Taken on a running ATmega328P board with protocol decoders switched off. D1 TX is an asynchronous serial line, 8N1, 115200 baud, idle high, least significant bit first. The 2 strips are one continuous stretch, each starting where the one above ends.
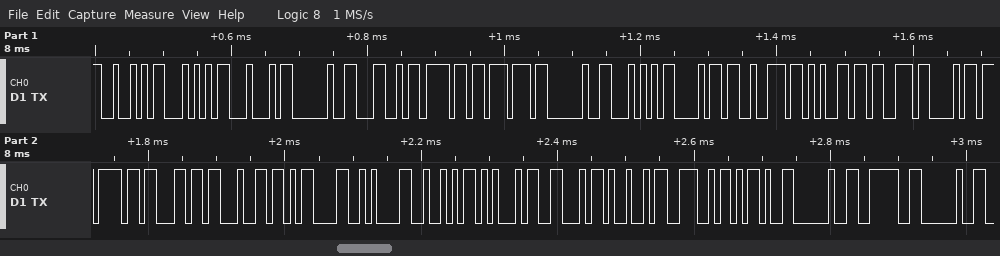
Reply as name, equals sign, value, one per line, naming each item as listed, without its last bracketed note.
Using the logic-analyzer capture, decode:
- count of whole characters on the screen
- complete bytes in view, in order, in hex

count of whole characters on the screen = 28
complete bytes in view, in order, in hex = 52 54 44 20 4C 6F 77 20 54 68 72 65 73 68 6F 6C 64 0D 0A 52 45 46 49 4E 2D 20 3E 20
